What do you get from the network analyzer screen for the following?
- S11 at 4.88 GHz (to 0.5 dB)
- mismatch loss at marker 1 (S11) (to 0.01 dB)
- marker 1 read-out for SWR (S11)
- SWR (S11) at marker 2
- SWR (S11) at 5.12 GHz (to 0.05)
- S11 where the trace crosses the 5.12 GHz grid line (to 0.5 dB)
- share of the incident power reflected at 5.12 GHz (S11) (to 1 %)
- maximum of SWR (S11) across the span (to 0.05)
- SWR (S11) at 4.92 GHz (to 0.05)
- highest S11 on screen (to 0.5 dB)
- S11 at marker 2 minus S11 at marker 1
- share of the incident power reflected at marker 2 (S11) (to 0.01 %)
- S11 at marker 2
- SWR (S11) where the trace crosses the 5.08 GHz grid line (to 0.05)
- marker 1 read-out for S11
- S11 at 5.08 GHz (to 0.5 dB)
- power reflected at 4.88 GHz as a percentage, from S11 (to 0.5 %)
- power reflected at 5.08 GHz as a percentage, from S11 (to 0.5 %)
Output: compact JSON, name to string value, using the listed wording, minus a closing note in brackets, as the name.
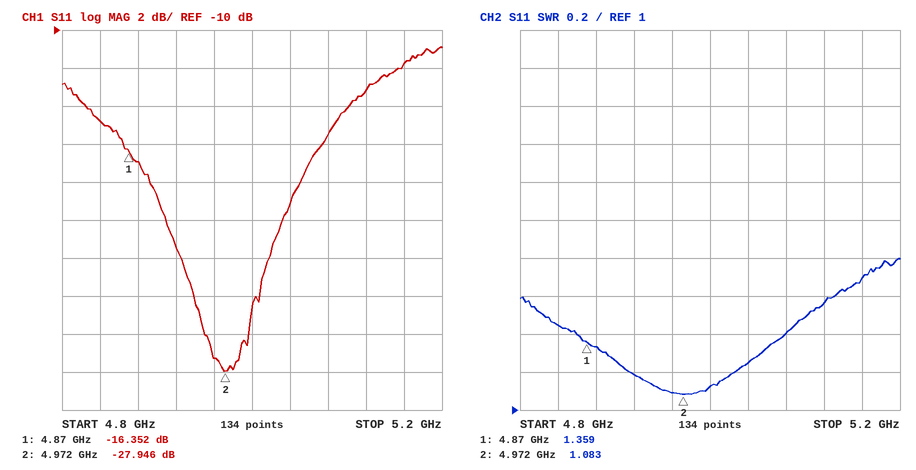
{"S11 at 4.88 GHz": "-17.0 dB", "mismatch loss at marker 1 (S11)": "0.10 dB", "marker 1 read-out for SWR": "1.359", "SWR (S11) at marker 2": "1.083", "SWR (S11) at 5.12 GHz": "1.55", "S11 where the trace crosses the 5.12 GHz grid line": "-13.0 dB", "share of the incident power reflected at 5.12 GHz (S11)": "5 %", "maximum of SWR (S11) across the span": "1.80", "SWR (S11) at 4.92 GHz": "1.20", "highest S11 on screen": "-11.0 dB", "S11 at marker 2 minus S11 at marker 1": "-11.594 dB", "share of the incident power reflected at marker 2 (S11)": "0.16 %", "S11 at marker 2": "-27.946 dB", "SWR (S11) where the trace crosses the 5.08 GHz grid line": "1.40", "marker 1 read-out for S11": "-16.352 dB", "S11 at 5.08 GHz": "-15.5 dB", "power reflected at 4.88 GHz as a percentage, from S11": "2.0 %", "power reflected at 5.08 GHz as a percentage, from S11": "3.0 %"}
